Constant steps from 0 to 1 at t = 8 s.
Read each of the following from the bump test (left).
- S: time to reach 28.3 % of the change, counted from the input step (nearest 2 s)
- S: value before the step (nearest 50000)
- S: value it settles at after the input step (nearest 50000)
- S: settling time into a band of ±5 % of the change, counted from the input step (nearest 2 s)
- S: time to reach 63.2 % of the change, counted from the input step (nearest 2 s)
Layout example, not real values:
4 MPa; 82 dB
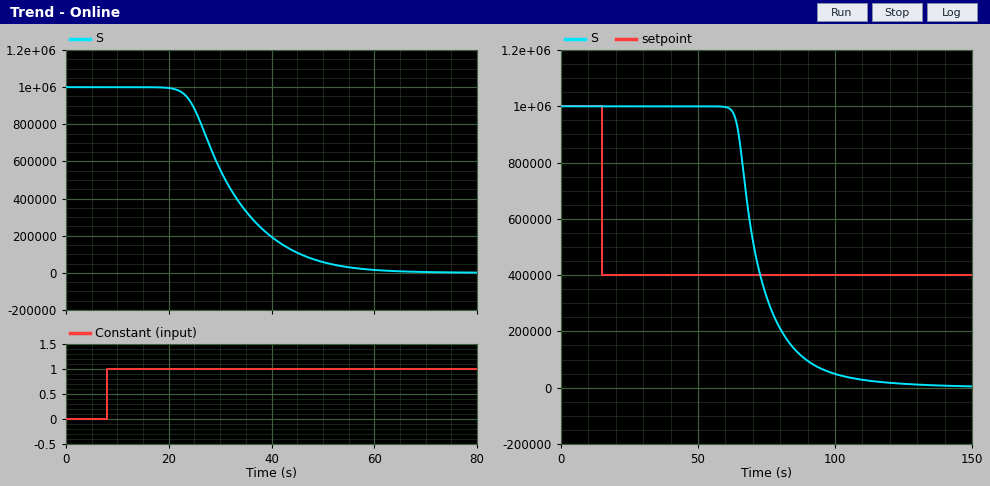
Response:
20 s; 1000000; 0; 44 s; 26 s
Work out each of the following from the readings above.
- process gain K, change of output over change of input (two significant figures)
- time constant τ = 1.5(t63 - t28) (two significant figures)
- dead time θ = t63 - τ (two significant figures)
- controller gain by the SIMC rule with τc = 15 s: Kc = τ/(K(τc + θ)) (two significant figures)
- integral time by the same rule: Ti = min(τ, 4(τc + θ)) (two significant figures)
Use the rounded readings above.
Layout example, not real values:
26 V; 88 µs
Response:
-1000000; 9.0 s; 17 s; -0.00000028; 9.0 s
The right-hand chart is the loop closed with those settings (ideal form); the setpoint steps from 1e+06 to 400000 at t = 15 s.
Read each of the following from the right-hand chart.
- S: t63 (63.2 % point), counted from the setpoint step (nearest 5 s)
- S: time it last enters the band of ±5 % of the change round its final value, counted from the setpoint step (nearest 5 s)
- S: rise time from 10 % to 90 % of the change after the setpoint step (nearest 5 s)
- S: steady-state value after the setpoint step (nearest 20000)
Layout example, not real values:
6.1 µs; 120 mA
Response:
60 s; 85 s; 25 s; 0
